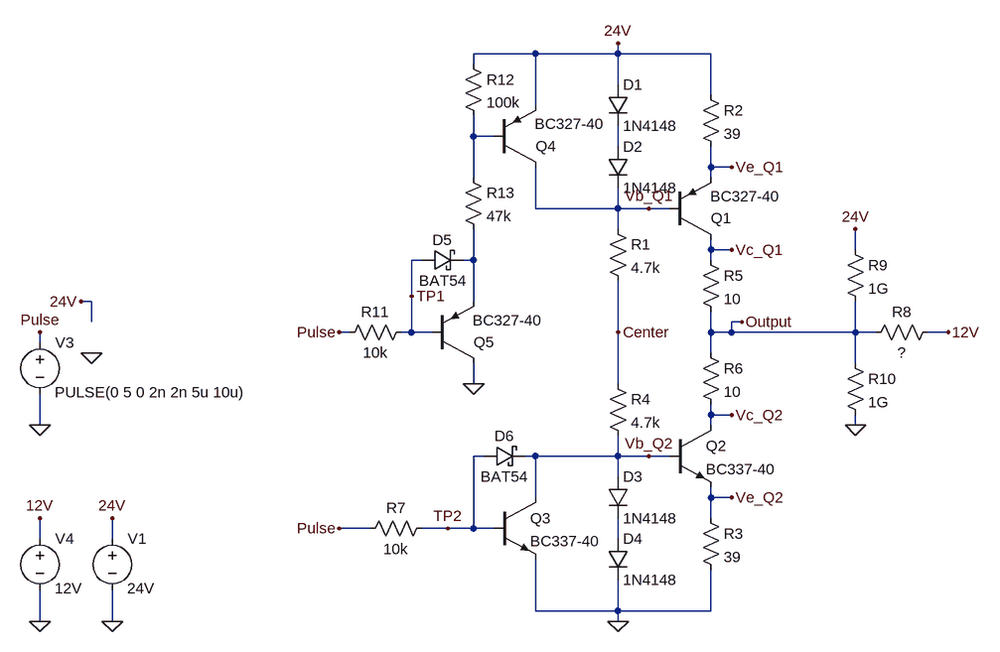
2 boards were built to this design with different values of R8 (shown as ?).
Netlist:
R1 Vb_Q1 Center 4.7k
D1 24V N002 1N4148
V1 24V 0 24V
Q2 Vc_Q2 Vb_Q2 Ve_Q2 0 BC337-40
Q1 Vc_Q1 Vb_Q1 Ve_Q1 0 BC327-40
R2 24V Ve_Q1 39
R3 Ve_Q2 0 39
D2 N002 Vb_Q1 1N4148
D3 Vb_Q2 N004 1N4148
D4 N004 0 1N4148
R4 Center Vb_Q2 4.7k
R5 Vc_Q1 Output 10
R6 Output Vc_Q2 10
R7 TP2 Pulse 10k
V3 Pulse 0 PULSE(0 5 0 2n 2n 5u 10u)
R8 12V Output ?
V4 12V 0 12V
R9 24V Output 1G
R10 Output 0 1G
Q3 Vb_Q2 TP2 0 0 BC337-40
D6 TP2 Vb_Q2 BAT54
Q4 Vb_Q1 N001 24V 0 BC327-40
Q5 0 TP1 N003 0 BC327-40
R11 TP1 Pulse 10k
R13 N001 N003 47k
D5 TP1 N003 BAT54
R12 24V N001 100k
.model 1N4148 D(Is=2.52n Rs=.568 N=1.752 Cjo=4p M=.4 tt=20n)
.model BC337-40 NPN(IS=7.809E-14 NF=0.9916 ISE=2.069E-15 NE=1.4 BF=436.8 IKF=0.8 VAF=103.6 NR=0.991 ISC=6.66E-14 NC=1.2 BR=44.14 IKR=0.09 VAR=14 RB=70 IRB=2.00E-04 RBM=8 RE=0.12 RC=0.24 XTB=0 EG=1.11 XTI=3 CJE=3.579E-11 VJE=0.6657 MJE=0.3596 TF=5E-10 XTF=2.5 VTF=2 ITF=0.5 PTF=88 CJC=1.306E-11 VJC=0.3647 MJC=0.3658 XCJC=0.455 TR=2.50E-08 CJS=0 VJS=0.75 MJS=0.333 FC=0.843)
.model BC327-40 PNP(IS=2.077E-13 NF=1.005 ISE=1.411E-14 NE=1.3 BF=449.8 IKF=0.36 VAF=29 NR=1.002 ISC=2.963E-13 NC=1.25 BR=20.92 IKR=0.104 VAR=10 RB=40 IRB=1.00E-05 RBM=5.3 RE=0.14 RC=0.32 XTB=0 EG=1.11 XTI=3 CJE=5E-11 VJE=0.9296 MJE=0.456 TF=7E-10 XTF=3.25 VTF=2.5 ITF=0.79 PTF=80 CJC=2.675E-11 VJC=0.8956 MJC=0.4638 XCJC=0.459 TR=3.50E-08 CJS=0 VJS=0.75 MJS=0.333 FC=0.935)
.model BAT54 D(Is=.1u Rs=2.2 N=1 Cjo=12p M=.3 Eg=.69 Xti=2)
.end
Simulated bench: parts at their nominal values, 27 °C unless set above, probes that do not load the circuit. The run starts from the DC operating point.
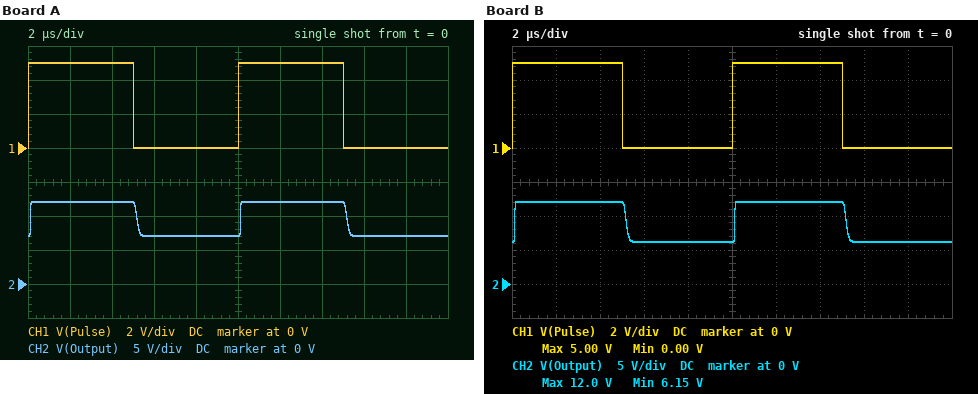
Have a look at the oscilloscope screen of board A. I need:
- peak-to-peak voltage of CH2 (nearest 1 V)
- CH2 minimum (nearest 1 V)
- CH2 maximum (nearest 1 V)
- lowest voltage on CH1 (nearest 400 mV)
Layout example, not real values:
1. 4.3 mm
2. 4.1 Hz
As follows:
1. 5 V
2. 7 V
3. 12 V
4. 0 V
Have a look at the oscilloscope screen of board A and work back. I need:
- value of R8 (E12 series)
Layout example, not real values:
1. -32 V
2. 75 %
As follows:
1. 330 Ω
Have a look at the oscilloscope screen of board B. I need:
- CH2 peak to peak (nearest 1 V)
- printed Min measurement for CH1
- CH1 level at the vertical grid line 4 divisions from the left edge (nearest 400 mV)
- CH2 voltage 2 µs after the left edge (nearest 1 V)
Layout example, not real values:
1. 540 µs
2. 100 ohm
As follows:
1. 6 V
2. 0.00 V
3. 0 V
4. 12 V
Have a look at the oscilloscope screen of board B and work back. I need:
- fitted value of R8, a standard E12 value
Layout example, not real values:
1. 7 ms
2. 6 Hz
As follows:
1. 390 Ω
